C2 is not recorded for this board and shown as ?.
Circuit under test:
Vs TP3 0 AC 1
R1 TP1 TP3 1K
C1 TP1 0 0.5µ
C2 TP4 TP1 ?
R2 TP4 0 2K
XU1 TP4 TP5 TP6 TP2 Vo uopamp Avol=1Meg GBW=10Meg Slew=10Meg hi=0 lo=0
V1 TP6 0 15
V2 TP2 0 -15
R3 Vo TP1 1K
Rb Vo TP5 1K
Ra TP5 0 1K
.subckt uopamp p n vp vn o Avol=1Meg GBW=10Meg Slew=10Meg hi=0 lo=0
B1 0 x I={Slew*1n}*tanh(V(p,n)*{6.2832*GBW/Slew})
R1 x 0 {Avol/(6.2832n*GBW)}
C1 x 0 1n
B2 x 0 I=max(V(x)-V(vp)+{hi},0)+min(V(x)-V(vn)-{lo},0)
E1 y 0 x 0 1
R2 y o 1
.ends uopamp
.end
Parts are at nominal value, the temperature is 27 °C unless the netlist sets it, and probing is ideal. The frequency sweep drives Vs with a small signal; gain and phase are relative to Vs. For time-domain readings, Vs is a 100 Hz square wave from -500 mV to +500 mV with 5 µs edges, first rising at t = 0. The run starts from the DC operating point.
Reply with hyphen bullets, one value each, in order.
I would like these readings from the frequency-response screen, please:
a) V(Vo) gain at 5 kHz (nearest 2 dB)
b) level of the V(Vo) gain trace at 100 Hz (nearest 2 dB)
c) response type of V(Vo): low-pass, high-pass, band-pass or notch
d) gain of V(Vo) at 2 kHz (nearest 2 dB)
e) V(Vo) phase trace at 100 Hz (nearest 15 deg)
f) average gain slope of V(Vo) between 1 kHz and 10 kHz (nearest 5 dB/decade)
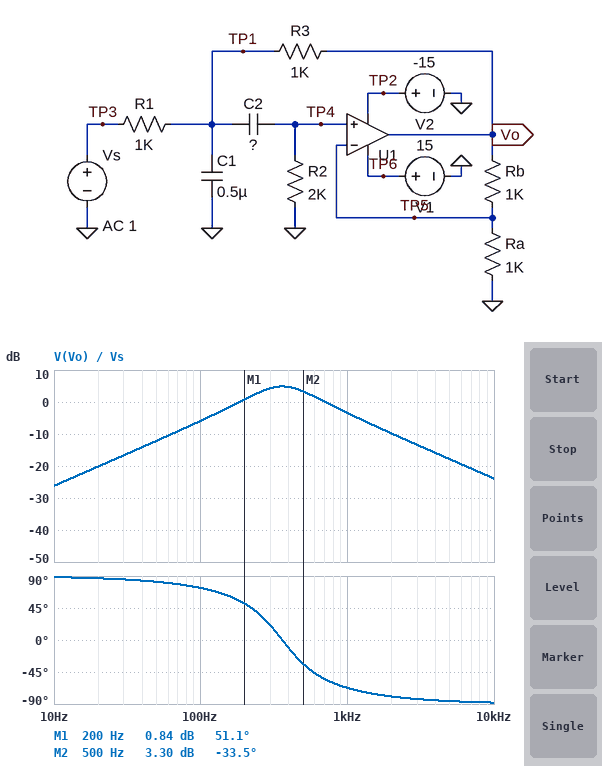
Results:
- -18 dB
- -6 dB
- band-pass
- -10 dB
- 75 deg
- -20 dB/decade
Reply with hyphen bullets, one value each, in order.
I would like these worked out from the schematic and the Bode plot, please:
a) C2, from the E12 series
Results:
- 390 nF
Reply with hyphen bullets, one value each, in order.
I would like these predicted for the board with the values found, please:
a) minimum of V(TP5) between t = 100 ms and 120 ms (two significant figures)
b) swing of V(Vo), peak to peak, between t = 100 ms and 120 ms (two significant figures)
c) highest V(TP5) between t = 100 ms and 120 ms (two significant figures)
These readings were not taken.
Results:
- -480 mV
- 1.9 V
- 480 mV
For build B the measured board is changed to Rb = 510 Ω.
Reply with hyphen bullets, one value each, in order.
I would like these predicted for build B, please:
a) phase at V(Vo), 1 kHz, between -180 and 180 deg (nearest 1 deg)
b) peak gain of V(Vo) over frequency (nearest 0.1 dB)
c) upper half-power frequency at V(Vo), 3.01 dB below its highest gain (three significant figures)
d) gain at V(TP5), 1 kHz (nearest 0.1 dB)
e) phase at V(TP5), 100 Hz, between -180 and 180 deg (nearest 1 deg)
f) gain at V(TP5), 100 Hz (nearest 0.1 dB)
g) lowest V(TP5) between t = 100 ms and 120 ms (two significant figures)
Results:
- -59 deg
- -0.7 dB
- 704 Hz
- -10.1 dB
- 67 deg
- -12.3 dB
- -400 mV
